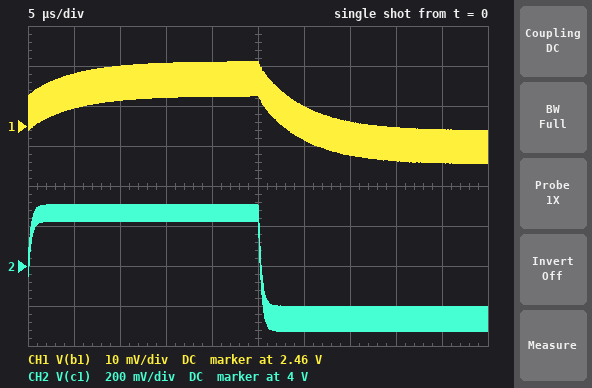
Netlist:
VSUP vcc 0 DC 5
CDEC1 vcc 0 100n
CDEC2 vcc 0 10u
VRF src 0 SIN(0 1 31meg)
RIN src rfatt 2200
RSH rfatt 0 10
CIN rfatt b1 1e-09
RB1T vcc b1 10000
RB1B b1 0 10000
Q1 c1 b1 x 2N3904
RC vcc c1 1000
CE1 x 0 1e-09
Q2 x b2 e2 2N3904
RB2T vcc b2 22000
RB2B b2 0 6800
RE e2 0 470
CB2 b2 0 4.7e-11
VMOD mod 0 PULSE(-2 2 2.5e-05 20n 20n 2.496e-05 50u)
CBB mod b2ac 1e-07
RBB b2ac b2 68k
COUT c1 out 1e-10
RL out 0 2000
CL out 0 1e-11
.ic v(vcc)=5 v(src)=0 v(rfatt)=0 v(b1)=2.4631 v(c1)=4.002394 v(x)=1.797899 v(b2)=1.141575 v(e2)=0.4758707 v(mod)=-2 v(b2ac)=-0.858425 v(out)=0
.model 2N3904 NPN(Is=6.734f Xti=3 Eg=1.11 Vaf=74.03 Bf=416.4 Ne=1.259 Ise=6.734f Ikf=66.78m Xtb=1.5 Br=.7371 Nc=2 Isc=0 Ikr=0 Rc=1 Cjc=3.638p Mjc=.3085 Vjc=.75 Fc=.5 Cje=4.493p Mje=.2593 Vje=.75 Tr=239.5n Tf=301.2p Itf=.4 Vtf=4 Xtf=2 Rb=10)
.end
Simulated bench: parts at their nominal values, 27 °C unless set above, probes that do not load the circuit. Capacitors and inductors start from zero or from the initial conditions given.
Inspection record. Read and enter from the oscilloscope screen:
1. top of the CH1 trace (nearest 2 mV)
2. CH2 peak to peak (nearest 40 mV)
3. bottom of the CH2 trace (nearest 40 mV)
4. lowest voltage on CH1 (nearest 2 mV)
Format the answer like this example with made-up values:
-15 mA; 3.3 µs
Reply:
2.476 V; 640 mV; 3.68 V; 2.450 V
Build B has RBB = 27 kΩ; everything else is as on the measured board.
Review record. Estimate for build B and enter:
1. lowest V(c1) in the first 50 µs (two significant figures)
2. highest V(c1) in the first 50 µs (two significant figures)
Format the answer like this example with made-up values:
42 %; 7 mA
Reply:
3.3 V; 4.6 V
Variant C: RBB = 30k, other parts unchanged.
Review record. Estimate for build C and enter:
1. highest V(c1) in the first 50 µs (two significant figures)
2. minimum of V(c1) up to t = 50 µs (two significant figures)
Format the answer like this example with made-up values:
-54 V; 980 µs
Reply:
4.6 V; 3.4 V
